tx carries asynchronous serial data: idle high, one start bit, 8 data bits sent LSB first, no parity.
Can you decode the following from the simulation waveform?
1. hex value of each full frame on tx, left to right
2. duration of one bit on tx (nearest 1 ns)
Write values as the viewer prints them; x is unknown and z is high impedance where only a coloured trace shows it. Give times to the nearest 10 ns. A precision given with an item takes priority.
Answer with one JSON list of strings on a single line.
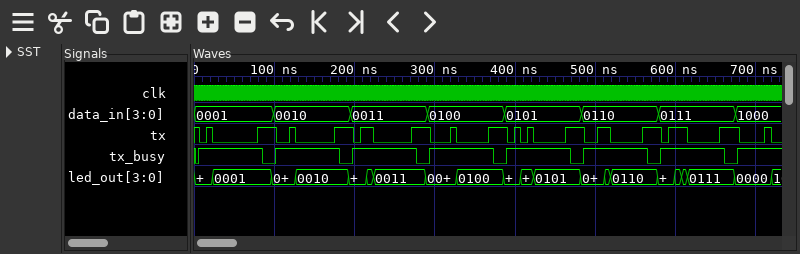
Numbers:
["01, 02, 03, 04, 05, 06, 07", "8 ns"]
